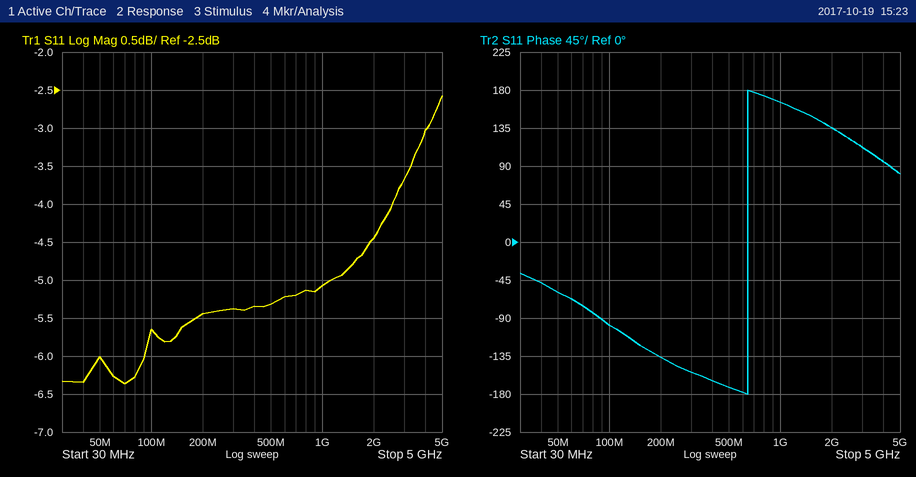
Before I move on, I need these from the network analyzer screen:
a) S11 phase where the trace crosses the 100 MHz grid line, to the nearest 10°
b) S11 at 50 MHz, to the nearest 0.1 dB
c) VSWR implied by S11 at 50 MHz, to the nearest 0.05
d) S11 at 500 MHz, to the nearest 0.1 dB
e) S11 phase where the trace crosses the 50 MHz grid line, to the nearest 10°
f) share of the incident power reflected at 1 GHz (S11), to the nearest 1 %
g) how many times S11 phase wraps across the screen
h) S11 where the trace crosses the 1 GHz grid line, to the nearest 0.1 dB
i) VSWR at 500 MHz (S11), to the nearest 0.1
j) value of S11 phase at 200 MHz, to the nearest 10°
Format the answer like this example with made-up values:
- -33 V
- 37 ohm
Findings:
- -100°
- -6.0 dB
- 3.00
- -5.3 dB
- -60°
- 31 %
- 1
- -5.1 dB
- 3.4
- -140°
